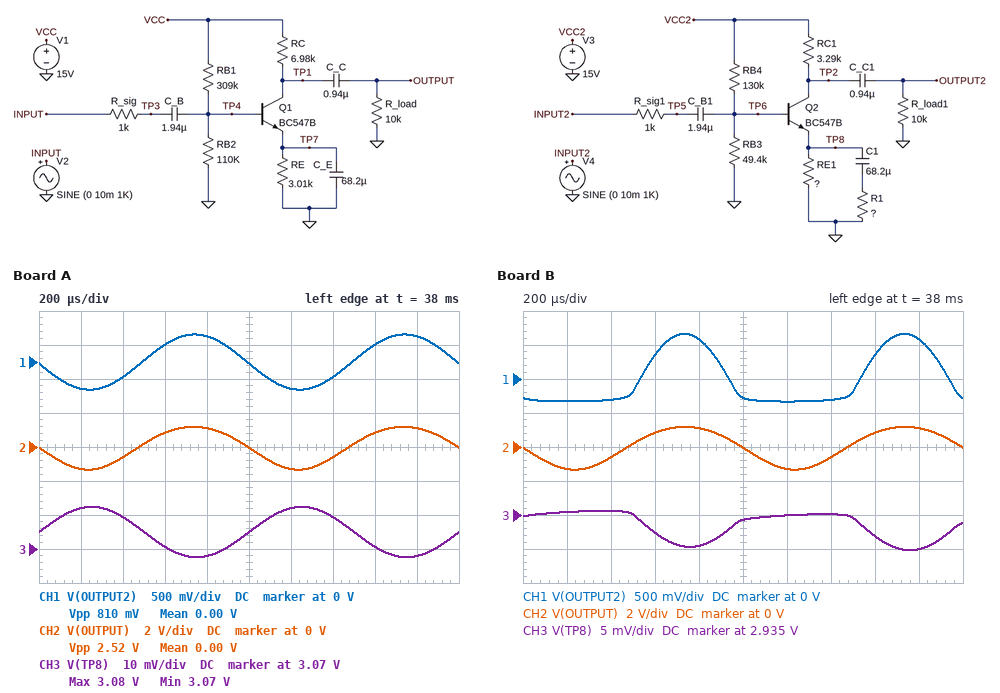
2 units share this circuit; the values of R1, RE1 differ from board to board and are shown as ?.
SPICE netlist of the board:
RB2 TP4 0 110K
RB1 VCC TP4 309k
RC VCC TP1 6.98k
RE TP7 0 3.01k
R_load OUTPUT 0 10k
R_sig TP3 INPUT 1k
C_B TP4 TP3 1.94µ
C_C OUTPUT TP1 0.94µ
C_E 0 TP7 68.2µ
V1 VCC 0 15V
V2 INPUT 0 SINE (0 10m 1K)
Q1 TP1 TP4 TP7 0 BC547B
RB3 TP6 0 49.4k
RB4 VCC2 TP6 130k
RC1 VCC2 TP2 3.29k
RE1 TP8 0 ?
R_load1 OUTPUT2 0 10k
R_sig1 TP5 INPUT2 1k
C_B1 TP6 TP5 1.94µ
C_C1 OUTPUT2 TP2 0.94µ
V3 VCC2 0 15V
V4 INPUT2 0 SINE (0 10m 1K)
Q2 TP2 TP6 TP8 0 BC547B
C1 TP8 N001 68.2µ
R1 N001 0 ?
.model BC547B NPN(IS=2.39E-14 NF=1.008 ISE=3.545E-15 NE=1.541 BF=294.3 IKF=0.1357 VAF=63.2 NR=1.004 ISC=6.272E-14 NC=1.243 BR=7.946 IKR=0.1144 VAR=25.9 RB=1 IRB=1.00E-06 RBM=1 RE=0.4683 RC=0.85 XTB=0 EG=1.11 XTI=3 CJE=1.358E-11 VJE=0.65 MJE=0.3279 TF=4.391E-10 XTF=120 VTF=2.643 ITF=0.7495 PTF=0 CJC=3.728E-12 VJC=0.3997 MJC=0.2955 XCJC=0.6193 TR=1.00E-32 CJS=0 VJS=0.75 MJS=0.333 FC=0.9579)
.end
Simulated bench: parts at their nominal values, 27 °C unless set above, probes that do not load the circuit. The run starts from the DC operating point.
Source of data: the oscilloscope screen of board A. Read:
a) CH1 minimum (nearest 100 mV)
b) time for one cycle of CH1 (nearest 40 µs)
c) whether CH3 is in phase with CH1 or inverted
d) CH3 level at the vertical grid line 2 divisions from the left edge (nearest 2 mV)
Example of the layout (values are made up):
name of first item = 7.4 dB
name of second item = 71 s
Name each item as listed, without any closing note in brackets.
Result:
CH1 minimum = -400 mV
time for one cycle of CH1 = 1.00 ms
whether CH3 is in phase with CH1 or inverted = inverted
CH3 level at the vertical grid line 2 divisions from the left edge = 3.080 V
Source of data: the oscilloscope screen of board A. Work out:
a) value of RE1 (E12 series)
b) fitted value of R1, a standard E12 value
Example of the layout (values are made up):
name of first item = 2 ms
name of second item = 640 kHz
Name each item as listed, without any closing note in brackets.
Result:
value of RE1 = 1 kΩ
fitted value of R1, a standard E12 value = 47 Ω
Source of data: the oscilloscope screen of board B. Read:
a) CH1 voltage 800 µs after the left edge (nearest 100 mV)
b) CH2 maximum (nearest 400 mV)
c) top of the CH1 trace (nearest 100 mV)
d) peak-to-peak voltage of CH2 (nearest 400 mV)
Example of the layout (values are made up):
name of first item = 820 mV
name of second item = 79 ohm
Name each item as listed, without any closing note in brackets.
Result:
CH1 voltage 800 µs after the left edge = 600 mV
CH2 maximum = 1.2 V
top of the CH1 trace = 700 mV
peak-to-peak voltage of CH2 = 2.4 V
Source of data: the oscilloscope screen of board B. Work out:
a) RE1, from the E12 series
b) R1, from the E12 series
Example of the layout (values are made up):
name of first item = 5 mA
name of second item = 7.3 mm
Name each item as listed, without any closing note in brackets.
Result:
RE1, from the E12 series = 820 Ω
R1, from the E12 series = 12 Ω
